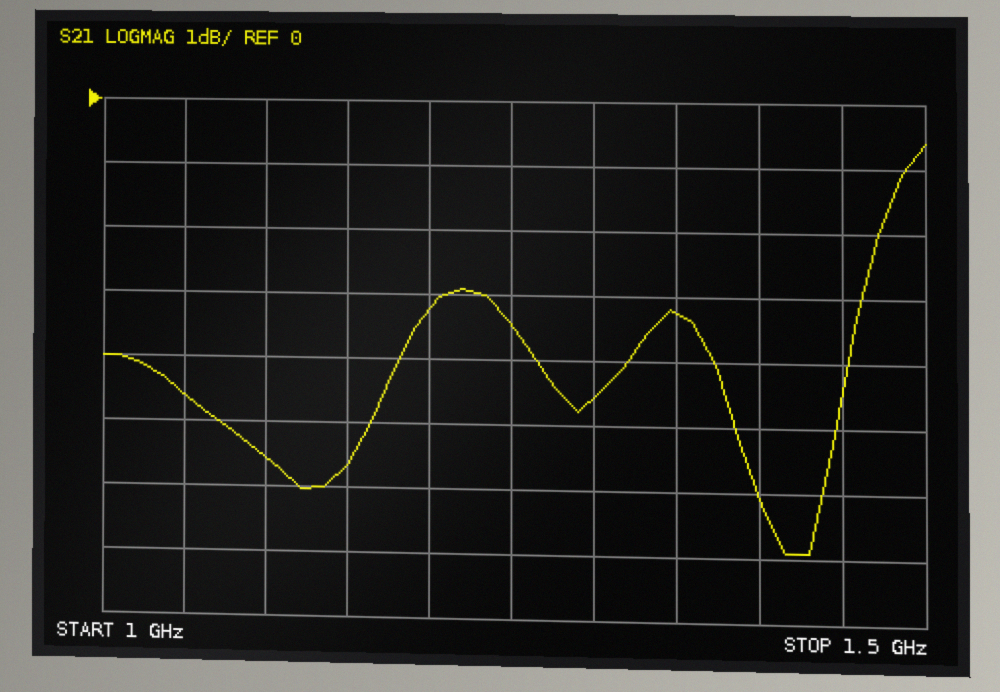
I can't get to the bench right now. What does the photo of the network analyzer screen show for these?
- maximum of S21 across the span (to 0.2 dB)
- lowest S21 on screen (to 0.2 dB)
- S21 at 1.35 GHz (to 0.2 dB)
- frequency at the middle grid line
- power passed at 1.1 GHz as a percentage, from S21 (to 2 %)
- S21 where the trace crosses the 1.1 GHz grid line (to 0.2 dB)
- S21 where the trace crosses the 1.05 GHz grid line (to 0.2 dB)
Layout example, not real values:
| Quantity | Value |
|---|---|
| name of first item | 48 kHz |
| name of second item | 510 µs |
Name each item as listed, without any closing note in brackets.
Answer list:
| Quantity | Value |
|---|---|
| maximum of S21 across the span | -0.6 dB |
| lowest S21 on screen | -7.0 dB |
| S21 at 1.35 GHz | -3.2 dB |
| frequency at the middle grid line | 1.25 GHz |
| power passed at 1.1 GHz as a percentage, from S21 | 28 % |
| S21 where the trace crosses the 1.1 GHz grid line | -5.6 dB |
| S21 where the trace crosses the 1.05 GHz grid line | -4.6 dB |
